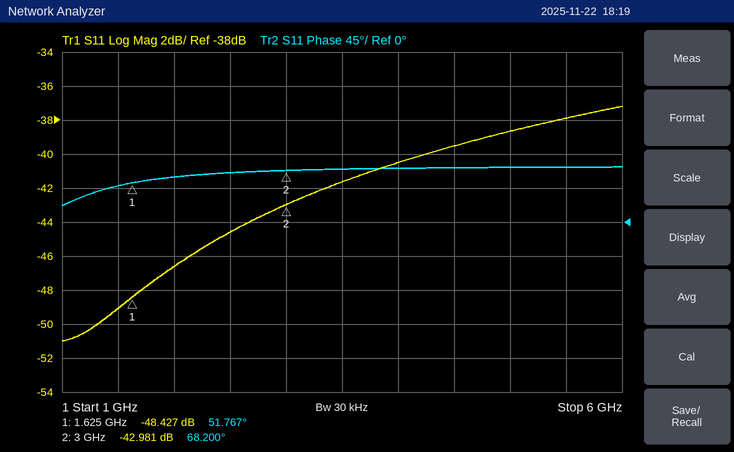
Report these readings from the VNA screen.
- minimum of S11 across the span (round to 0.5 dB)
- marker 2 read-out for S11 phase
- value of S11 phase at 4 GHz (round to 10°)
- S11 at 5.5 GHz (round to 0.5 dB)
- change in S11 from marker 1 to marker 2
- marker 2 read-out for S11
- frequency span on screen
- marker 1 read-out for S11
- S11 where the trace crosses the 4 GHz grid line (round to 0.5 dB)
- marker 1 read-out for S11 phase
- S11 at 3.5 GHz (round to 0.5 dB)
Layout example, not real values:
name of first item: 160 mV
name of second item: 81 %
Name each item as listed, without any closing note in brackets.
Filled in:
minimum of S11 across the span: -51.0 dB
marker 2 read-out for S11 phase: 68.200°
value of S11 phase at 4 GHz: 70°
S11 at 5.5 GHz: -38.0 dB
change in S11 from marker 1 to marker 2: 5.446 dB
marker 2 read-out for S11: -42.981 dB
frequency span on screen: 5 GHz
marker 1 read-out for S11: -48.427 dB
S11 where the trace crosses the 4 GHz grid line: -40.5 dB
marker 1 read-out for S11 phase: 51.767°
S11 at 3.5 GHz: -41.5 dB
